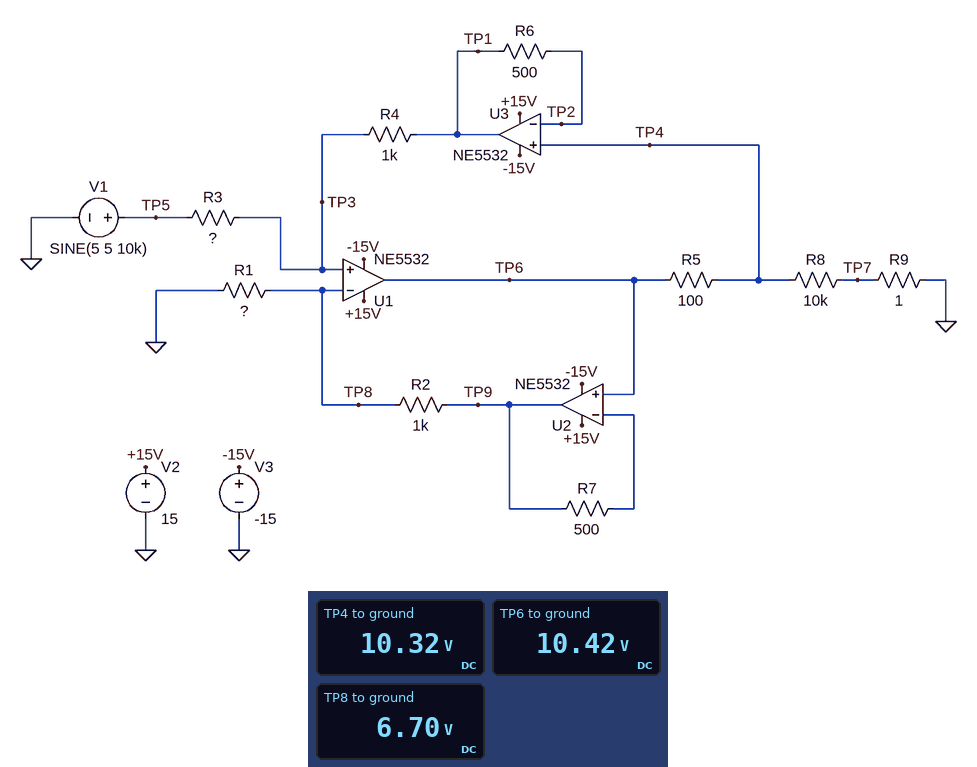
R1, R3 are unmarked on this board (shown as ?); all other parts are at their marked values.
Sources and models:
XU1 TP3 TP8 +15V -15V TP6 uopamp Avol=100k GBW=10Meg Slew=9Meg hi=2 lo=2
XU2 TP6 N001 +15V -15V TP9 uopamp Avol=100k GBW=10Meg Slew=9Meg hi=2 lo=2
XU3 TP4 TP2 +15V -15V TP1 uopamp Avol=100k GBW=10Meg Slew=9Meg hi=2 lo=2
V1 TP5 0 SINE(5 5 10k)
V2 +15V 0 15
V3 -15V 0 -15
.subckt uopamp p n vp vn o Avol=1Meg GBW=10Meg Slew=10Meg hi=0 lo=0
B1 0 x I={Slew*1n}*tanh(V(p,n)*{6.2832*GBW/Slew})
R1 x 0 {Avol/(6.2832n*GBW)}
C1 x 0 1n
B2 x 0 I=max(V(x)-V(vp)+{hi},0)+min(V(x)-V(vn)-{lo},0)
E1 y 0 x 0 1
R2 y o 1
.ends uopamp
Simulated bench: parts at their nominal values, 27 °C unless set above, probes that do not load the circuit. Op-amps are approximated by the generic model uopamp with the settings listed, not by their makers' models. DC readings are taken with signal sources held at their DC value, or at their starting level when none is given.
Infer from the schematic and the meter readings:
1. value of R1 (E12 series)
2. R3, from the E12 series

1.8 kΩ
470 Ω
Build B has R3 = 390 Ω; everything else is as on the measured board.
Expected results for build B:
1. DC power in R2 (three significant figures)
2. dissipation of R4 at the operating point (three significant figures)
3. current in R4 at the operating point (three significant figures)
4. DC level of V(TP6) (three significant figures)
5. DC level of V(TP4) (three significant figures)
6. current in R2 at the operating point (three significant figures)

12.4 mW
11.7 mW
3.42 mA
9.85 V
9.76 V
3.52 mA
